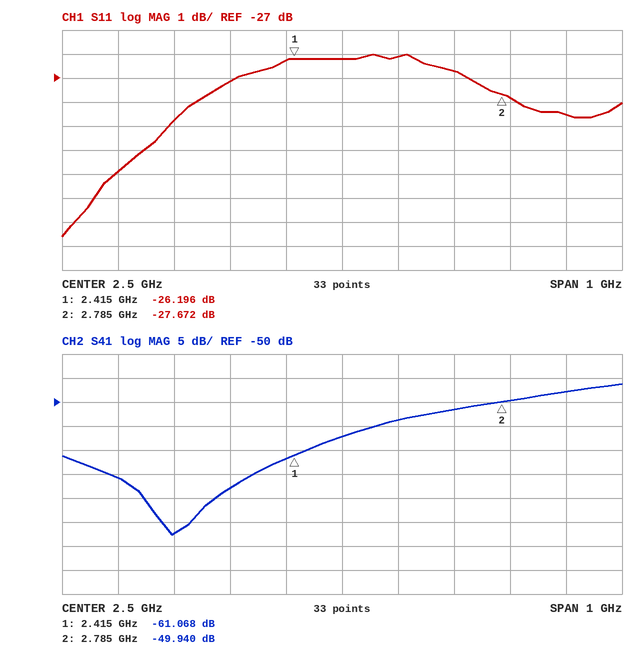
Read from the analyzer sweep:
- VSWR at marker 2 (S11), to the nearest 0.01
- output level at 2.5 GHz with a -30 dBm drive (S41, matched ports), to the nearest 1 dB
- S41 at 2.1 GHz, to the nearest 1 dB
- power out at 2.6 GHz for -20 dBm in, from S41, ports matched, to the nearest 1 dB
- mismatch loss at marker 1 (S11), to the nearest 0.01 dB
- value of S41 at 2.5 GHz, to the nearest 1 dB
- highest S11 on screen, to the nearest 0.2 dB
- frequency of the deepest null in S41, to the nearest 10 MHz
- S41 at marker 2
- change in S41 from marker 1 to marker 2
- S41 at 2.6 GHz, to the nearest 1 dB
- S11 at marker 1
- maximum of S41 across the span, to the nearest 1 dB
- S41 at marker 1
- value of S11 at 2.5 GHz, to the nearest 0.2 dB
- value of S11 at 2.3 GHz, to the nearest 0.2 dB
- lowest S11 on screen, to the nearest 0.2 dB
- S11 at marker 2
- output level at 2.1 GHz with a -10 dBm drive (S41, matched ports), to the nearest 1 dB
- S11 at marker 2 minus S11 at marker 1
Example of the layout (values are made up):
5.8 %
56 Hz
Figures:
1.09
-87 dBm
-66 dB
-74 dBm
0.01 dB
-57 dB
-26.0 dB
2.20 GHz
-49.940 dB
11.128 dB
-54 dB
-26.196 dB
-46 dB
-61.068 dB
-26.2 dB
-27.2 dB
-33.6 dB
-27.672 dB
-76 dBm
-1.476 dB
